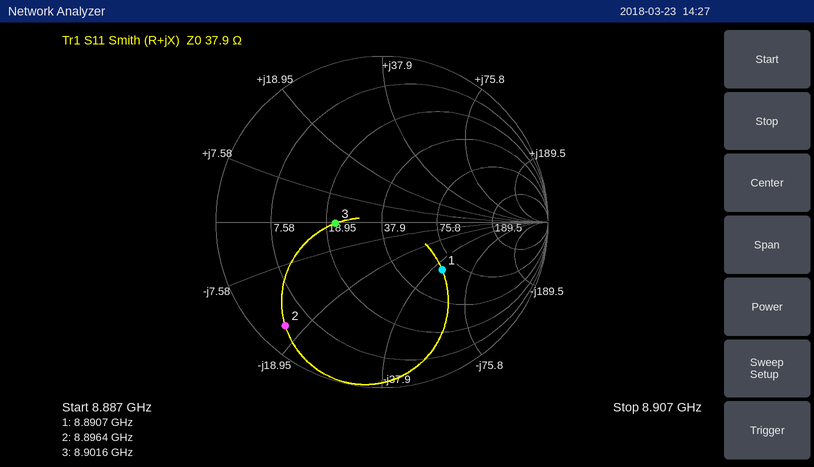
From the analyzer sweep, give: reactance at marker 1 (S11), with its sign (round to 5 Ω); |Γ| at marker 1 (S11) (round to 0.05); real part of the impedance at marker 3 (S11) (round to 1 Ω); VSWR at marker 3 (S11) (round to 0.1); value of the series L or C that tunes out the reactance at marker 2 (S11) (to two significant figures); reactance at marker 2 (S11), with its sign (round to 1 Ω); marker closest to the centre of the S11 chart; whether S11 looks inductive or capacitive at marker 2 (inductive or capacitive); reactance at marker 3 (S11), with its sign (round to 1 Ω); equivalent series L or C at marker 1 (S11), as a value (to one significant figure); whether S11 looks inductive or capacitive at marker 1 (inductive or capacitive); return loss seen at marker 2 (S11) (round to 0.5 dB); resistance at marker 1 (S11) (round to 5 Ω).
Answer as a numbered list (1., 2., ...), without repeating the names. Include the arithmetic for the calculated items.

1. -45 Ω
2. 0.45
3. 21 Ω
4. 1.8
5. L = 16 Ω/(2π × 8.8964 GHz) ≈ 286 pH, so 290 pH to two significant figures
6. -16 Ω
7. marker 3
8. capacitive
9. 0 Ω
10. C = 1/(2π × 8.8907 GHz × 45 Ω) ≈ 398 fF, so 400 fF to one significant figure
11. capacitive
12. 1.5 dB
13. 60 Ω
